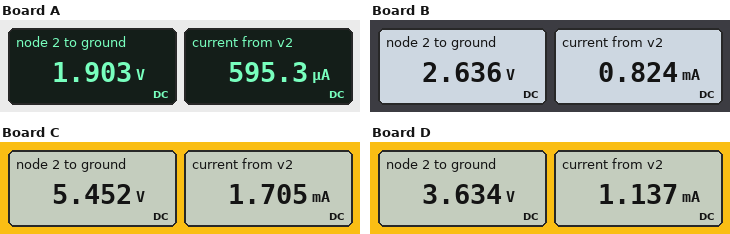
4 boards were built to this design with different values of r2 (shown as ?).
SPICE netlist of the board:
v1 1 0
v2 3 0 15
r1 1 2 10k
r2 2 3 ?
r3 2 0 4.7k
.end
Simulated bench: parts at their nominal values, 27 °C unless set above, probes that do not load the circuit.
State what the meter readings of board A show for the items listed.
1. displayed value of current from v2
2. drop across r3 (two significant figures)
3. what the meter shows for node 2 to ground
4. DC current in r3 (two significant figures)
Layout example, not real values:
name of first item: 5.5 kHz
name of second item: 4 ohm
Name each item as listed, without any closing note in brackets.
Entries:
displayed value of current from v2: 595.3 µA
drop across r3: 1.9 V
what the meter shows for node 2 to ground: 1.903 V
DC current in r3: 400 µA
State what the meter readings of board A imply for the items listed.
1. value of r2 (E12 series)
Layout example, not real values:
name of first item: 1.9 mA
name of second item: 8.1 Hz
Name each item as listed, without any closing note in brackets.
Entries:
value of r2: 22 kΩ
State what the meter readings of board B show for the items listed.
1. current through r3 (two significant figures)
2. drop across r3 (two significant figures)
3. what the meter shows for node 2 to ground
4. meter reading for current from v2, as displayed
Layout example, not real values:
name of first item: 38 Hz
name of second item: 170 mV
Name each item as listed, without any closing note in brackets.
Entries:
current through r3: 560 µA
drop across r3: 2.6 V
what the meter shows for node 2 to ground: 2.636 V
meter reading for current from v2, as displayed: 0.824 mA
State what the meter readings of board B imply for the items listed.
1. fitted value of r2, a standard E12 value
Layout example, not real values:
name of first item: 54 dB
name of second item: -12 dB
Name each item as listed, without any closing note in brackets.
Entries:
fitted value of r2, a standard E12 value: 15 kΩ
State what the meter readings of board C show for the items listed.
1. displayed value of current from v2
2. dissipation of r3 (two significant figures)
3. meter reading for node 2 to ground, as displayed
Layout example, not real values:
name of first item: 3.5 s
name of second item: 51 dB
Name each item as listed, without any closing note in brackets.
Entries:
displayed value of current from v2: 1.705 mA
dissipation of r3: 6.3 mW
meter reading for node 2 to ground, as displayed: 5.452 V
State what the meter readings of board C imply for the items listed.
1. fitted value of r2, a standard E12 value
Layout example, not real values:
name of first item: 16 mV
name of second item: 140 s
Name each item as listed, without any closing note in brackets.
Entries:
fitted value of r2, a standard E12 value: 5.6 kΩ
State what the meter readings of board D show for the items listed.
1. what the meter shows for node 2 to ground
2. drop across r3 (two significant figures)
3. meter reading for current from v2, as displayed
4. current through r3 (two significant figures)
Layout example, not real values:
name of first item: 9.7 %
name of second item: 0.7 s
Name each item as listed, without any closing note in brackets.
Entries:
what the meter shows for node 2 to ground: 3.634 V
drop across r3: 3.6 V
meter reading for current from v2, as displayed: 1.137 mA
current through r3: 770 µA
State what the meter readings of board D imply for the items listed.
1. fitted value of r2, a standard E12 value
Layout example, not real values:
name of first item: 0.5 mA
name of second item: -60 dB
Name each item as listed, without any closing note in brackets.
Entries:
fitted value of r2, a standard E12 value: 10 kΩ
